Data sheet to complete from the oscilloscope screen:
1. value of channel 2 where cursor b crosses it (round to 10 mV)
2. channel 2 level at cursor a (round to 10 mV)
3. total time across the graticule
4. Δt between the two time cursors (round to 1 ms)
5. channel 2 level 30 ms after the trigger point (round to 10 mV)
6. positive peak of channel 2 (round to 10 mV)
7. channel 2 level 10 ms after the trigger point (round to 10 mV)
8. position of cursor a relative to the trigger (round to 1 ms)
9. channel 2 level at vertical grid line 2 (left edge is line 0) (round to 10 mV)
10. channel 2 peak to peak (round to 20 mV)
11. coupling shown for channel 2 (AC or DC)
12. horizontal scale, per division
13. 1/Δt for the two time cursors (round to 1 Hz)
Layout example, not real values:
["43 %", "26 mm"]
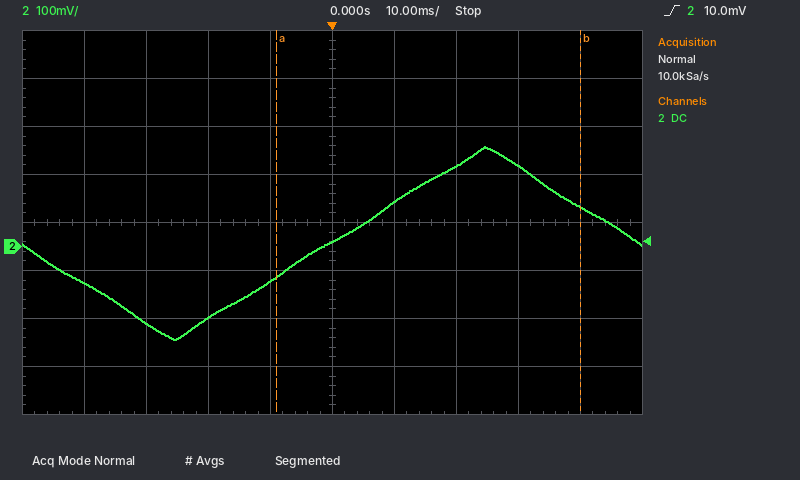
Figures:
["80 mV", "-60 mV", "100 ms", "49 ms", "170 mV", "210 mV", "90 mV", "-9 ms", "-160 mV", "400 mV", "DC", "10 ms", "20 Hz"]
